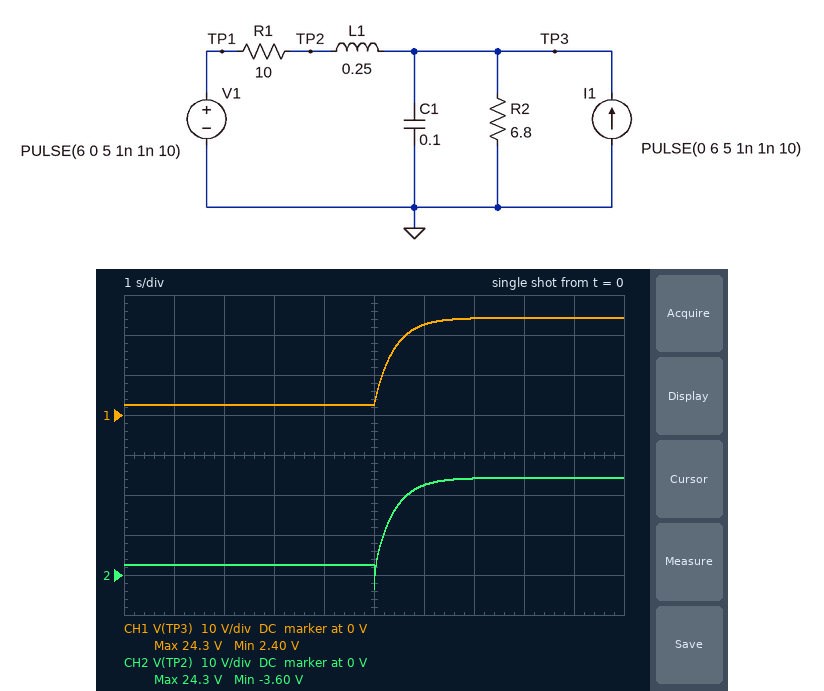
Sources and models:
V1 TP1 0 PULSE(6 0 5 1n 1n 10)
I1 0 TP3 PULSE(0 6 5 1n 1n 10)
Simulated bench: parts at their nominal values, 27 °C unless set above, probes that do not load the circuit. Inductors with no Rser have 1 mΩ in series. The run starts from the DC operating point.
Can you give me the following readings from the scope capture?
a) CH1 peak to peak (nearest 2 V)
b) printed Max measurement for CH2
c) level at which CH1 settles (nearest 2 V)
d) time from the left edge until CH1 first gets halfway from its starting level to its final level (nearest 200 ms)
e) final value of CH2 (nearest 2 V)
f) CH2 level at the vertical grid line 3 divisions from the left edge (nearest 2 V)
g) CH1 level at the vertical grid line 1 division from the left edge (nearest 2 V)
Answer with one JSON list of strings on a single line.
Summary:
["22 V", "24.3 V", "24 V", "5.2 s", "24 V", "2 V", "2 V"]
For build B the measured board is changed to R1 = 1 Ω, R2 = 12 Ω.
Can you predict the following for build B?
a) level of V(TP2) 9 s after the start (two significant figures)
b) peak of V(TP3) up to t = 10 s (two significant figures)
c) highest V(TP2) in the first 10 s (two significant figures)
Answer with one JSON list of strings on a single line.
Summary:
["5.5 V", "11 V", "7.7 V"]
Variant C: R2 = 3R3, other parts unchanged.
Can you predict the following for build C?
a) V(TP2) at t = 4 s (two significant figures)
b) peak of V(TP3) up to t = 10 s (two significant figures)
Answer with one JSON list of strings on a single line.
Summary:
["1.5 V", "15 V"]
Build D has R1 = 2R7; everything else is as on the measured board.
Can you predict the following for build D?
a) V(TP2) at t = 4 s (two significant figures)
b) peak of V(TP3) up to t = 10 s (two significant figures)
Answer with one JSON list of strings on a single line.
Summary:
["4.3 V", "12 V"]
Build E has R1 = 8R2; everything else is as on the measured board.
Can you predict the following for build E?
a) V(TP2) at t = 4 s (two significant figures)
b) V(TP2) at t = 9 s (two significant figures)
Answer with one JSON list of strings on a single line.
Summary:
["2.7 V", "22 V"]
